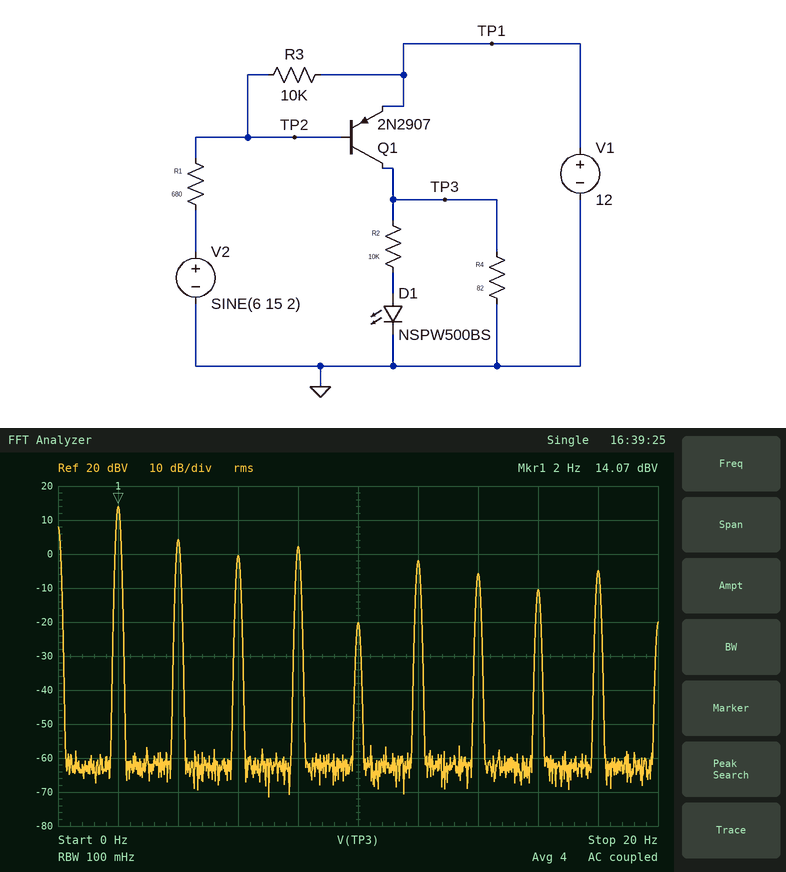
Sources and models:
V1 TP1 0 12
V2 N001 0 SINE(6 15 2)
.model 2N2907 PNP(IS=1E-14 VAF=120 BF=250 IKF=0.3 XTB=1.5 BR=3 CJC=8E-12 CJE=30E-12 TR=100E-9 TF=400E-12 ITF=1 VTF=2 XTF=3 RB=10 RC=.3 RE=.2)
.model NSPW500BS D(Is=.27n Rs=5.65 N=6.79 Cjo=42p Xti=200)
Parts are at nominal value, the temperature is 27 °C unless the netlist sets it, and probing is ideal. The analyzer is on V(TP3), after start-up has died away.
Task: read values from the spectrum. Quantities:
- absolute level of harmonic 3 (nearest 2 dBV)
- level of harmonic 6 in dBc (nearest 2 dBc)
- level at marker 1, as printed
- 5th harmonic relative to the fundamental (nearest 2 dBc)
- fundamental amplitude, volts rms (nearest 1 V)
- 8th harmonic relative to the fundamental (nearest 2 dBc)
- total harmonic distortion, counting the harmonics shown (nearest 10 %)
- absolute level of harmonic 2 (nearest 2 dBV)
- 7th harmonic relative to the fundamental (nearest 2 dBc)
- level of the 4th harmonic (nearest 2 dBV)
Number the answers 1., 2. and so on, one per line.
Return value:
1. 0 dBV
2. -16 dBc
3. 14.07 dBV
4. -34 dBc
5. 5 V
6. -24 dBc
7. 50 %
8. 4 dBV
9. -20 dBc
10. 2 dBV
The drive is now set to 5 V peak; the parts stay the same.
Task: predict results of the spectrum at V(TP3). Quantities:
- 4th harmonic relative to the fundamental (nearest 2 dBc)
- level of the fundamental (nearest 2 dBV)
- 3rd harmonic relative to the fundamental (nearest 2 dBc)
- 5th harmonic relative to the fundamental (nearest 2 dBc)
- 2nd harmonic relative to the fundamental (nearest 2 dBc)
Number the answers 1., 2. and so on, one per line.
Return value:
1. -2 dBc
2. 0 dBV
3. -2 dBc
4. -4 dBc
5. 0 dBc
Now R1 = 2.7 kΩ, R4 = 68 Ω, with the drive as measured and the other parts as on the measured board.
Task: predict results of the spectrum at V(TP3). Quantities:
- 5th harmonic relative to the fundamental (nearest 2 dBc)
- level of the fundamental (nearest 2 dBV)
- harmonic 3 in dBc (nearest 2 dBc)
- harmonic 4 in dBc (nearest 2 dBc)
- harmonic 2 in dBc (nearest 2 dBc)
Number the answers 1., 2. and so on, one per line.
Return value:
1. -24 dBc
2. 14 dBV
3. -12 dBc
4. -14 dBc
5. -12 dBc
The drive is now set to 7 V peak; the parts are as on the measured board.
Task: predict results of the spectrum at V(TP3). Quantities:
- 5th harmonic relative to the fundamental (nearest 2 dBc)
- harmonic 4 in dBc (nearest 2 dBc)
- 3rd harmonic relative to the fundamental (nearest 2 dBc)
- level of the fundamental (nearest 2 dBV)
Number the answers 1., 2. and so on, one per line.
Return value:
1. -14 dBc
2. -40 dBc
3. -10 dBc
4. 12 dBV
